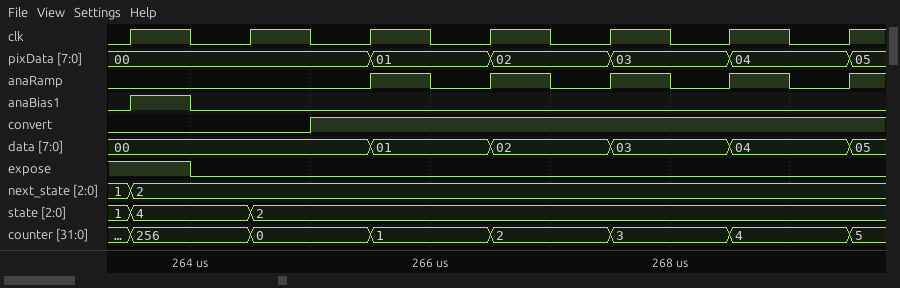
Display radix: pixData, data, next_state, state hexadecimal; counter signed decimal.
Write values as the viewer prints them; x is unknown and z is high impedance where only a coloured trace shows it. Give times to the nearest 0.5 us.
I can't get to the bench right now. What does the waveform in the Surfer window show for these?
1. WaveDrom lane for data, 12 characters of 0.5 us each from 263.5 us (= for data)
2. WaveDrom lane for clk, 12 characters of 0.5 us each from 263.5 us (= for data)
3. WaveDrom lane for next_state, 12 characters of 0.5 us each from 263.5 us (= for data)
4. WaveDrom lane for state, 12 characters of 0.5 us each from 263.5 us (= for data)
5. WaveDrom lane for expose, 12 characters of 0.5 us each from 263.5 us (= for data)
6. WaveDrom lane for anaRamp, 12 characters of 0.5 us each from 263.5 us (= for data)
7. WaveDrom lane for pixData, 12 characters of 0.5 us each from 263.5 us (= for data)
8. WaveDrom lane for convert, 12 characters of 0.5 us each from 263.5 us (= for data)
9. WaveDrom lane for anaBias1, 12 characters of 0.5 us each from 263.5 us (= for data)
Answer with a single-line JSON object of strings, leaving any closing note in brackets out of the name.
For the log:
{"WaveDrom lane for data, 12 characters of 0.5 us each from 263.5 us": "{name: 'data', wave: '=...=.=.=.=.', data: '00 01 02 03 04'}", "WaveDrom lane for clk, 12 characters of 0.5 us each from 263.5 us": "{name: 'clk', wave: '101010101010'}", "WaveDrom lane for next_state, 12 characters of 0.5 us each from 263.5 us": "{name: 'next_state', wave: '=...........', data: '2'}", "WaveDrom lane for state, 12 characters of 0.5 us each from 263.5 us": "{name: 'state', wave: '=.=.........', data: '4 2'}", "WaveDrom lane for expose, 12 characters of 0.5 us each from 263.5 us": "{name: 'expose', wave: '10..........'}", "WaveDrom lane for anaRamp, 12 characters of 0.5 us each from 263.5 us": "{name: 'anaRamp', wave: '0...10101010'}", "WaveDrom lane for pixData, 12 characters of 0.5 us each from 263.5 us": "{name: 'pixData', wave: '=...=.=.=.=.', data: '00 01 02 03 04'}", "WaveDrom lane for convert, 12 characters of 0.5 us each from 263.5 us": "{name: 'convert', wave: '0..1........'}", "WaveDrom lane for anaBias1, 12 characters of 0.5 us each from 263.5 us": "{name: 'anaBias1', wave: '10..........'}"}
